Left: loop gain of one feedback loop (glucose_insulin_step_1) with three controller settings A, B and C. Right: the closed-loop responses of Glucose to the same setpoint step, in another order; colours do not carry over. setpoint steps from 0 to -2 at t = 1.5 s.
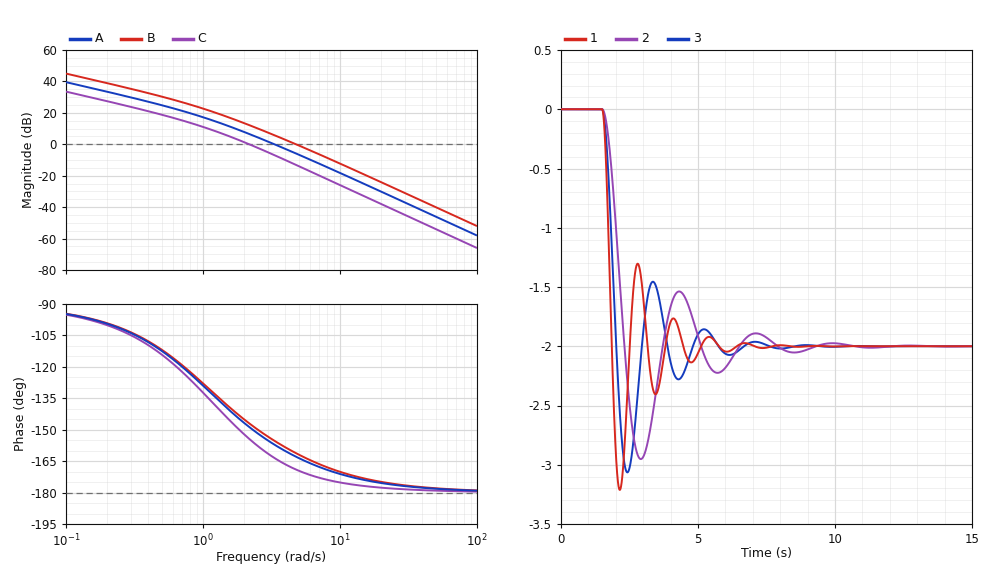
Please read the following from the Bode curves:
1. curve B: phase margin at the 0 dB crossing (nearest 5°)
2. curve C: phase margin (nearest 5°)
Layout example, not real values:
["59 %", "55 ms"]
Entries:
["20°", "25°"]
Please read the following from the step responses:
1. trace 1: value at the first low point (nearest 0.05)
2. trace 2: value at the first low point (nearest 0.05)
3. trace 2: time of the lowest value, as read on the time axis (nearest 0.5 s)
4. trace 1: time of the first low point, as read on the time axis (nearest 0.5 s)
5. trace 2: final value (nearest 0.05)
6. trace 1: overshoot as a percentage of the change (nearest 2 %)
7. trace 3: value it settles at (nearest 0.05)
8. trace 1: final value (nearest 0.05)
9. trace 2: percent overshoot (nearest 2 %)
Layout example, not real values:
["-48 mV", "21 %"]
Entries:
["-3.20", "-2.95", "3.0 s", "2.0 s", "-2.00", "60 %", "-2.00", "-2.00", "48 %"]
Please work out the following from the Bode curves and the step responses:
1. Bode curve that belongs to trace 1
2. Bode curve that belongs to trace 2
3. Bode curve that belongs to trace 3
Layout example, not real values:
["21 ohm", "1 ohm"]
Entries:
["B", "C", "A"]
